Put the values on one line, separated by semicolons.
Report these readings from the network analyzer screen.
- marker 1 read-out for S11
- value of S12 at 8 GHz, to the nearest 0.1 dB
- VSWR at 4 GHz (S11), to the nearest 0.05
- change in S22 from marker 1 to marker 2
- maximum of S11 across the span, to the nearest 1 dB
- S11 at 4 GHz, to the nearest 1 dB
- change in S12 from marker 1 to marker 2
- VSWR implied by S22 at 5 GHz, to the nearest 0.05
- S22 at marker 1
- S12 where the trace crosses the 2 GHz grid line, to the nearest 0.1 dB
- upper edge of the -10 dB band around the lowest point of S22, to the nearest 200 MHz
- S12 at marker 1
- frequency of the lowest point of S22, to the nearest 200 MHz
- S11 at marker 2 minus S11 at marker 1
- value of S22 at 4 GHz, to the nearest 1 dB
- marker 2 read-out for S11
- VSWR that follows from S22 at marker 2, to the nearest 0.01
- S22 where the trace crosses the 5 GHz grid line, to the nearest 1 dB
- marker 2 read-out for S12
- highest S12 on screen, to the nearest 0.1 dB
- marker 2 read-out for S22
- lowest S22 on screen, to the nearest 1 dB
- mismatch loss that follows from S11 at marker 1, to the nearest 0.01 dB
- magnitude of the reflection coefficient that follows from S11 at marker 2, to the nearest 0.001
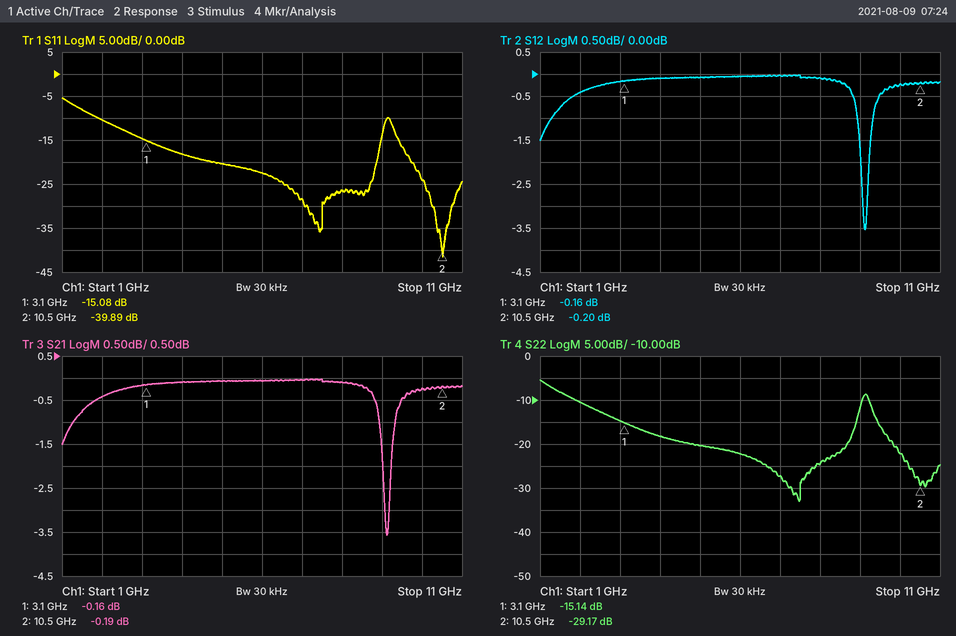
-15.08 dB; -0.1 dB; 1.30; -14.03 dB; -5 dB; -18 dB; -0.04 dB; 1.20; -15.14 dB; -0.4 dB; 9.0 GHz; -0.16 dB; 7.4 GHz; -24.81 dB; -18 dB; -39.89 dB; 1.07; -20 dB; -0.20 dB; 0.0 dB; -29.17 dB; -33 dB; 0.14 dB; 0.010
